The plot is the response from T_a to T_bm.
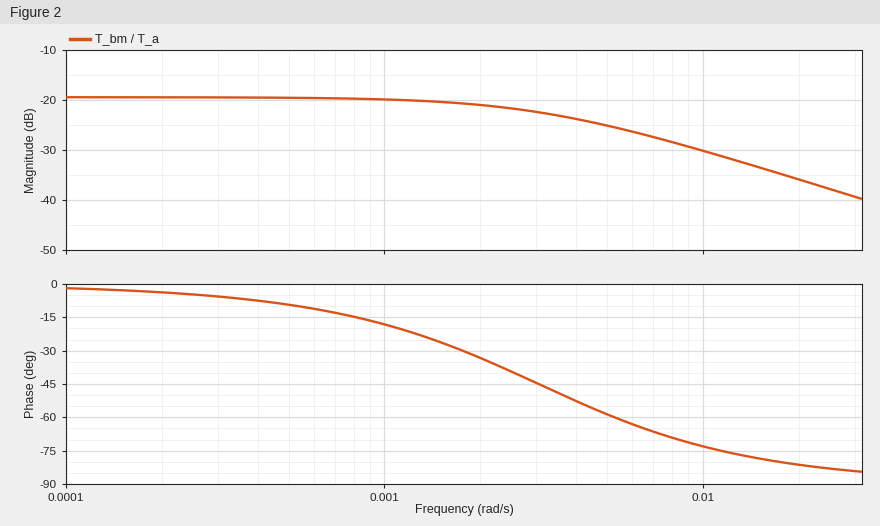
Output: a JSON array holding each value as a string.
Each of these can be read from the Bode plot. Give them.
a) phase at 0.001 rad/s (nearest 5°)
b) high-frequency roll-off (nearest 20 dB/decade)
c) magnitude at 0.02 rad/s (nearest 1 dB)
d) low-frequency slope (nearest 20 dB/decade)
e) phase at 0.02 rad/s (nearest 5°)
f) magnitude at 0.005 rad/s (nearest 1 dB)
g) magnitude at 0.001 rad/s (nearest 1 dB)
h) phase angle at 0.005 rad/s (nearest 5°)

["-20°", "-20 dB/decade", "-36 dB", "0 dB/decade", "-80°", "-25 dB", "-20 dB", "-60°"]
